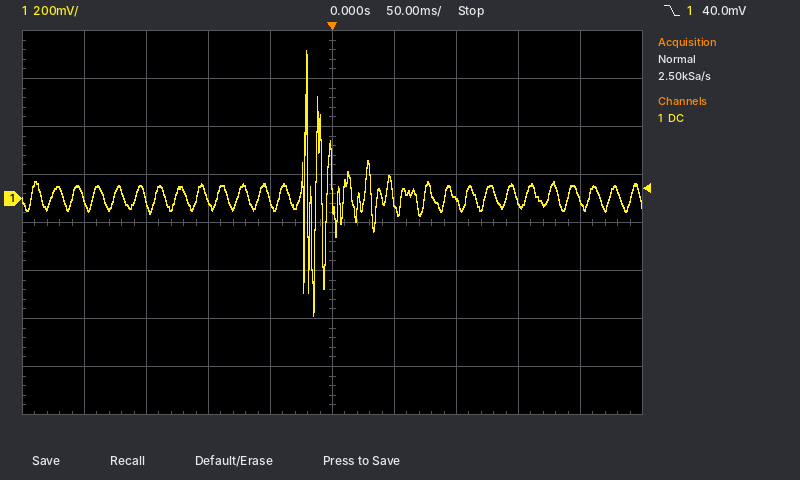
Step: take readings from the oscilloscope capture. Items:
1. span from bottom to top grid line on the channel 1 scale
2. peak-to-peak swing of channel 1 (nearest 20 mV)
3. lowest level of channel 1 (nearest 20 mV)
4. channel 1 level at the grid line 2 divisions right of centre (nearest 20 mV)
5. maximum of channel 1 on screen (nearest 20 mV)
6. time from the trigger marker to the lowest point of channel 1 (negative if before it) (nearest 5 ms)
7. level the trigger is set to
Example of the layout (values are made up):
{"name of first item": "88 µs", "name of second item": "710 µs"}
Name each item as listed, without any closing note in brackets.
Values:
{"span from bottom to top grid line on the channel 1 scale": "1.6 V", "peak-to-peak swing of channel 1": "1.10 V", "lowest level of channel 1": "-480 mV", "channel 1 level at the grid line 2 divisions right of centre": "0 mV", "maximum of channel 1 on screen": "620 mV", "time from the trigger marker to the lowest point of channel 1 (negative if before it)": "-15 ms", "level the trigger is set to": "40.0 mV"}
